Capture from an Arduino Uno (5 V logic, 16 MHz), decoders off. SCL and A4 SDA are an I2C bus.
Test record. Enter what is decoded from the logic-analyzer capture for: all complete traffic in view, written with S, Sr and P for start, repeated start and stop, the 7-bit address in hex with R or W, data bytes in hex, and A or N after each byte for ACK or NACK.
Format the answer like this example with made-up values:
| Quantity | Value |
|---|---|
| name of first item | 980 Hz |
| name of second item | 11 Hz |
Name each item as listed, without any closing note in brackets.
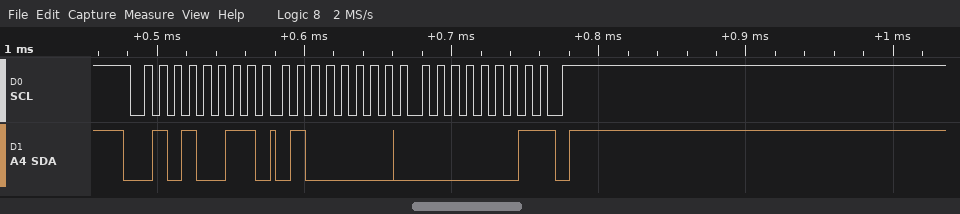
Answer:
| Quantity | Value |
|---|---|
| all complete traffic in view, written with S, Sr and P for start, repeated start and stop, the 7-bit address in hex with R or W, data bytes in hex, and A or N after each byte for ACK or NACK | S 29R A 40 A 01 N P |
